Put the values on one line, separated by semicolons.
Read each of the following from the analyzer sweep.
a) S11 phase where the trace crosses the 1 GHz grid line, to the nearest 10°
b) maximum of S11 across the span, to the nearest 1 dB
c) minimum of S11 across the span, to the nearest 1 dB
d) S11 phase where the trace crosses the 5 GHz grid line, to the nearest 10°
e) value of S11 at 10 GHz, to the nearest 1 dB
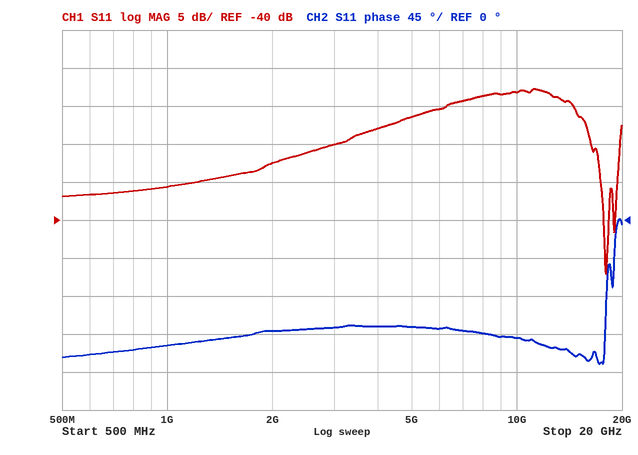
-150°; -23 dB; -47 dB; -130°; -23 dB
